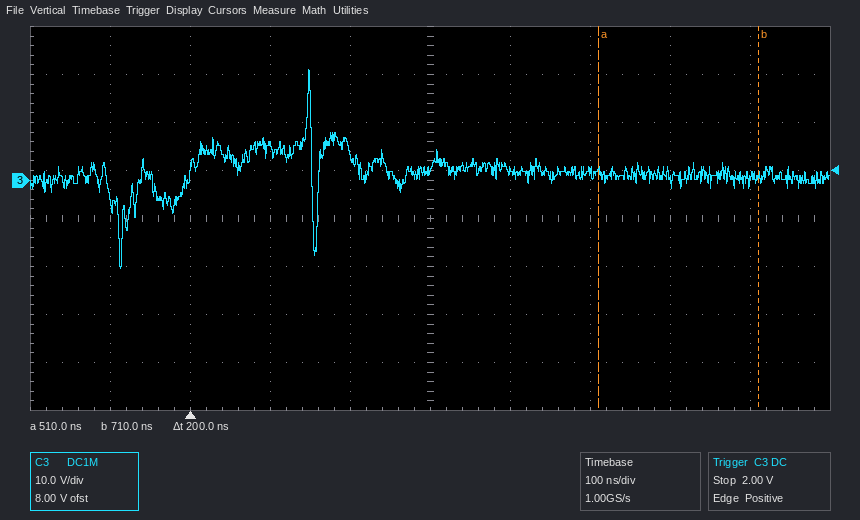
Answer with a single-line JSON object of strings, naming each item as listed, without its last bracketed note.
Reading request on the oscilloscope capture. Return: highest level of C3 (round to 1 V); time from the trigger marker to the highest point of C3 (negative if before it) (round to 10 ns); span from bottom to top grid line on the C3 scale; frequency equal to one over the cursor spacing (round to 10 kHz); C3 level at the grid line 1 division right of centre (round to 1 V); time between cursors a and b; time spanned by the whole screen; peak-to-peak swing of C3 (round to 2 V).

{"highest level of C3": "23 V", "time from the trigger marker to the highest point of C3 (negative if before it)": "+150 ns", "span from bottom to top grid line on the C3 scale": "80 V", "frequency equal to one over the cursor spacing": "5.00 MHz", "C3 level at the grid line 1 division right of centre": "2 V", "time between cursors a and b": "200 ns", "time spanned by the whole screen": "1 µs", "peak-to-peak swing of C3": "42 V"}
